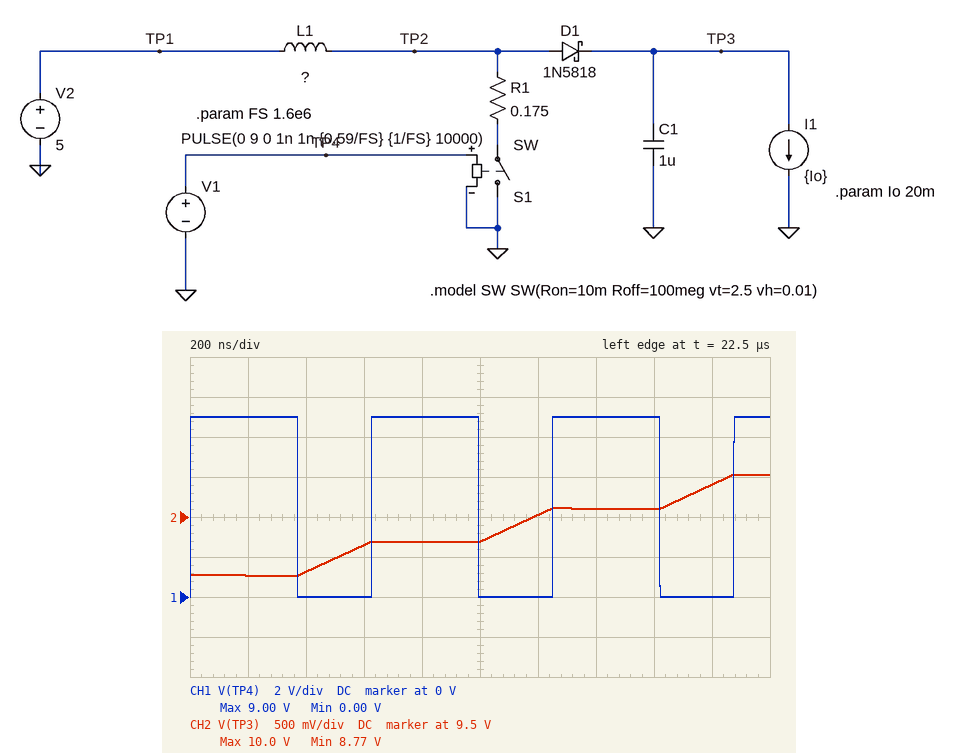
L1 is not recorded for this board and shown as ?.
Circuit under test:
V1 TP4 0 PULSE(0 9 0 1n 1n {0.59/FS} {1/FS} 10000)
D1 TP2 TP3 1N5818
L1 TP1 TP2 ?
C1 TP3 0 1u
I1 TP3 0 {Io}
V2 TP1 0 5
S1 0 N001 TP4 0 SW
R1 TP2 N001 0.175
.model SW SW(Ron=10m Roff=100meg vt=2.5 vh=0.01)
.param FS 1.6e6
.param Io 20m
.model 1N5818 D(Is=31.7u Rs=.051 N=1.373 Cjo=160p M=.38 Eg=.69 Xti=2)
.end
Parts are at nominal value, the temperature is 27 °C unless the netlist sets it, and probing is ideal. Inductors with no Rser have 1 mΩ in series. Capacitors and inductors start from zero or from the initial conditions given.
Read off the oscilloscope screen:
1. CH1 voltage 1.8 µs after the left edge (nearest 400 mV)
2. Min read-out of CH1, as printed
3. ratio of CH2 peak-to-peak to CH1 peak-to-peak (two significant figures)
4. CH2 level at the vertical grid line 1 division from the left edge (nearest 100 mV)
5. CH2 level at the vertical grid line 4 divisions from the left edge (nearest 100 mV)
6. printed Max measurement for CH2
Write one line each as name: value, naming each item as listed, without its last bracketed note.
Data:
CH1 voltage 1.8 µs after the left edge: 0 V
Min read-out of CH1, as printed: 0.00 V
ratio of CH2 peak-to-peak to CH1 peak-to-peak: 0.14
CH2 level at the vertical grid line 1 division from the left edge: 8.8 V
CH2 level at the vertical grid line 4 divisions from the left edge: 9.2 V
printed Max measurement for CH2: 10.0 V
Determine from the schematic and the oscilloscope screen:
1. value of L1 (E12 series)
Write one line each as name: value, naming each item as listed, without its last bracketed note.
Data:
value of L1: 47 µH
